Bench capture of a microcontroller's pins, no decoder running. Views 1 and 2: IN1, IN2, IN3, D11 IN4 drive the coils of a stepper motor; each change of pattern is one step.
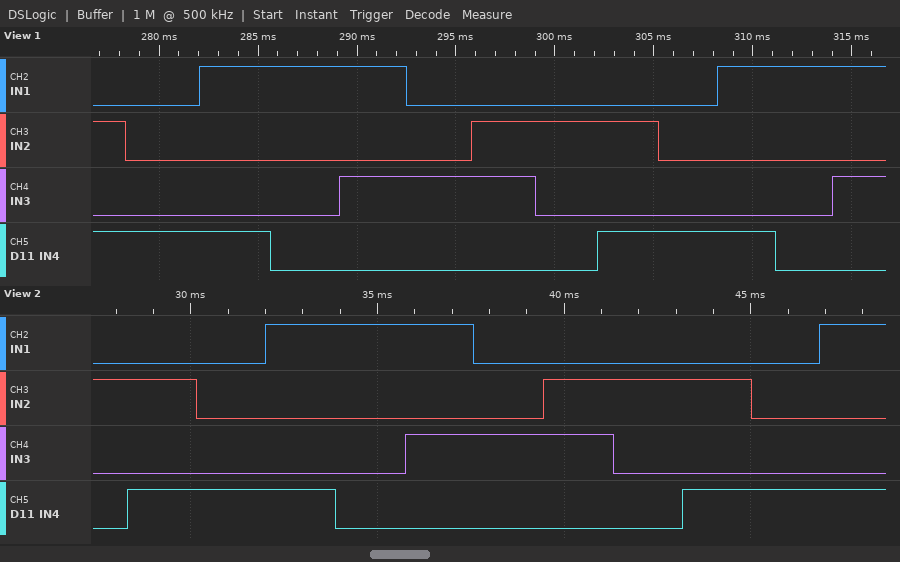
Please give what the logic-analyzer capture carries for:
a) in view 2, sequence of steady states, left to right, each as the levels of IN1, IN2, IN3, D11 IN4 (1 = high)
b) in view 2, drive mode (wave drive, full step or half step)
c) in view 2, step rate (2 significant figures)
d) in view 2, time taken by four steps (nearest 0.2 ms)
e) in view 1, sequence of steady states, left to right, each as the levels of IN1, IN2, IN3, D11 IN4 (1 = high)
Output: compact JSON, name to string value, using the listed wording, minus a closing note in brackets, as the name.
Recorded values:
{"in view 2, sequence of steady states, left to right, each as the levels of IN1, IN2, IN3, D11 IN4": "0100 0101 0001 1001 1000 1010 0010 0110 0100 0101 0001 1001", "in view 2, drive mode": "half step", "in view 2, step rate": "540 steps/s", "in view 2, time taken by four steps": "7.4 ms", "in view 1, sequence of steady states, left to right, each as the levels of IN1, IN2, IN3, D11 IN4": "0101 0001 1001 1000 1010 0010 0110 0100 0101 0001 1001 1000 1010"}
